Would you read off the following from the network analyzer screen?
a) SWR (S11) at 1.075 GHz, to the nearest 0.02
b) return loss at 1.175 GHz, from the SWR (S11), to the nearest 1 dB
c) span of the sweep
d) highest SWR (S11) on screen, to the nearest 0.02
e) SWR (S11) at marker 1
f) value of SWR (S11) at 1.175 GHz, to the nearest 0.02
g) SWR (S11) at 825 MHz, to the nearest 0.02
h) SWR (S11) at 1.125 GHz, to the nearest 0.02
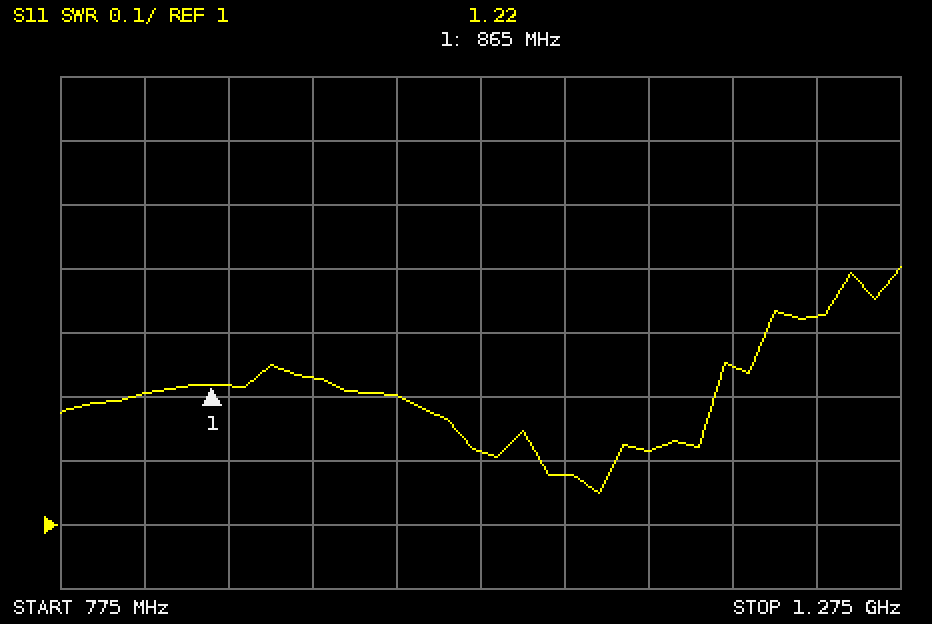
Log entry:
1.08
19 dB
500 MHz
1.40
1.22
1.24
1.20
1.12
